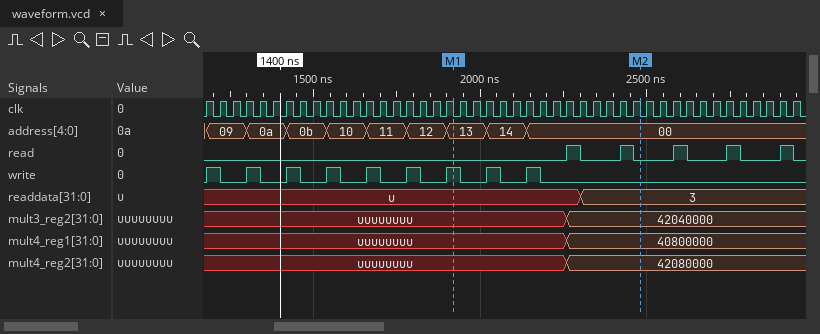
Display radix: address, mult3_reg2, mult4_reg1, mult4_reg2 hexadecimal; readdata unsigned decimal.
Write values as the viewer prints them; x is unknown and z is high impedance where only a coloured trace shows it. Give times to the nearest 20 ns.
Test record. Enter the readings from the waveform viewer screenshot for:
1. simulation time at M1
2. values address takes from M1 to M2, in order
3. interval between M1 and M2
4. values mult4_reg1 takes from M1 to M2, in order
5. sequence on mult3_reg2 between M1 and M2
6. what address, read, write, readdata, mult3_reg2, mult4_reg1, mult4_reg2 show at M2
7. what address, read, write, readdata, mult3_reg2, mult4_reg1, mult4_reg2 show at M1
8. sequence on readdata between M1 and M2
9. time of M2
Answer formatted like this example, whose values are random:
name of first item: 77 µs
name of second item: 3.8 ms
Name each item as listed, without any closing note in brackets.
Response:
simulation time at M1: 1920 ns
values address takes from M1 to M2, in order: 13, 14, 00
interval between M1 and M2: 560 ns
values mult4_reg1 takes from M1 to M2, in order: uuuuuuuu, 40800000
sequence on mult3_reg2 between M1 and M2: uuuuuuuu, 42040000
what address, read, write, readdata, mult3_reg2, mult4_reg1, mult4_reg2 show at M2: address=00, read=0, write=0, readdata=3, mult3_reg2=42040000, mult4_reg1=40800000, mult4_reg2=42080000
what address, read, write, readdata, mult3_reg2, mult4_reg1, mult4_reg2 show at M1: address=13, read=0, write=1, readdata=u, mult3_reg2=uuuuuuuu, mult4_reg1=uuuuuuuu, mult4_reg2=uuuuuuuu
sequence on readdata between M1 and M2: u, 3
time of M2: 2480 ns
